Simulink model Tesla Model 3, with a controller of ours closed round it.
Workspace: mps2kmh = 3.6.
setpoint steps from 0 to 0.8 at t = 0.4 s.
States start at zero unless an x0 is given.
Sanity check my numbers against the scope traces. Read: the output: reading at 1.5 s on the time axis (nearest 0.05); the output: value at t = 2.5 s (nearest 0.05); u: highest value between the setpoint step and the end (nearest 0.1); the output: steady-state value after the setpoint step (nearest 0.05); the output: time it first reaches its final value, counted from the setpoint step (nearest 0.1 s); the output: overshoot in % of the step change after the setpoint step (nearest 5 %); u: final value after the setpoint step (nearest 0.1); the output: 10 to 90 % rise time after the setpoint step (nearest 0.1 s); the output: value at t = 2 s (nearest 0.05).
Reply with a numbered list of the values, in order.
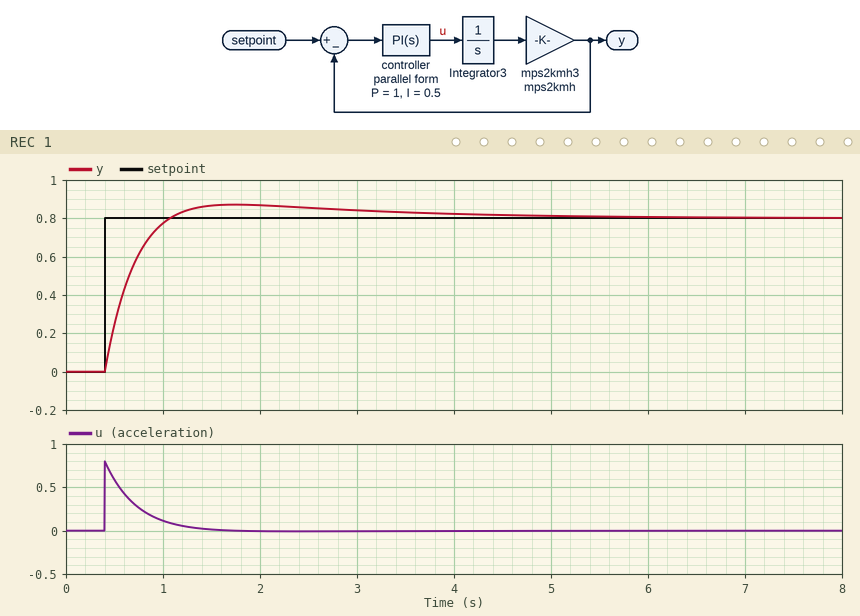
1. 0.85
2. 0.85
3. 0.8
4. 0.80
5. 0.7 s
6. 10 %
7. 0.0
8. 0.5 s
9. 0.85
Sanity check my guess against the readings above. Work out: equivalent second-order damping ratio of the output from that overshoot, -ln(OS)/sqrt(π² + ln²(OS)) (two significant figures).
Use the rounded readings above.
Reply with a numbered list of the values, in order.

1. 0.59
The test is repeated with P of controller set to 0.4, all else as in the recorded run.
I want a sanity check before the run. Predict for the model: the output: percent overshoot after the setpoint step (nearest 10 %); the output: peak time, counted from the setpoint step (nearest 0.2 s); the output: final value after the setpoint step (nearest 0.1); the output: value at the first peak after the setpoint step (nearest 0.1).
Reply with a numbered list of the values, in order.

1. 30 %
2. 1.8 s
3. 0.8
4. 1.0
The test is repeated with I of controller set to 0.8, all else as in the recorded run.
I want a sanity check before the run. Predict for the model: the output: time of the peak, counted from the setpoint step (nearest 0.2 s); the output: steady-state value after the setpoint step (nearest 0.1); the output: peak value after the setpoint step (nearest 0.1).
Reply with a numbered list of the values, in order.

1. 1.2 s
2. 0.8
3. 0.9
